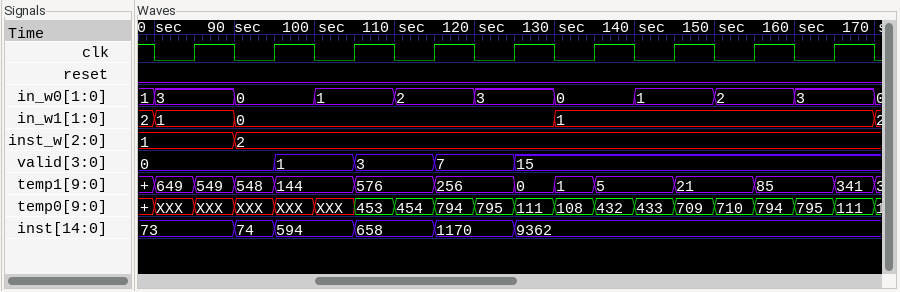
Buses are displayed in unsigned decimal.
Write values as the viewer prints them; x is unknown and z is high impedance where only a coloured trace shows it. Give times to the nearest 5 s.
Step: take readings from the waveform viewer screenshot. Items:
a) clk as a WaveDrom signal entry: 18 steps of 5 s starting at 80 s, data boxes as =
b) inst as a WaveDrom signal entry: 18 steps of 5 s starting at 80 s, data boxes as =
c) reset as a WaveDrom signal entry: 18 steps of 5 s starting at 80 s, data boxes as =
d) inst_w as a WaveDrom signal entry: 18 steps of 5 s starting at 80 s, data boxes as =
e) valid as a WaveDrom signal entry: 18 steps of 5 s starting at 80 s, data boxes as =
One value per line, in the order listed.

{name: 'clk', wave: '010101010101010101'}
{name: 'inst', wave: '=.==.=.=.=........', data: '73 74 594 658 1170 9362'}
{name: 'reset', wave: '0.................'}
{name: 'inst_w', wave: '=.=...............', data: '1 2'}
{name: 'valid', wave: '=..=.=.=.=........', data: '0 1 3 7 15'}
